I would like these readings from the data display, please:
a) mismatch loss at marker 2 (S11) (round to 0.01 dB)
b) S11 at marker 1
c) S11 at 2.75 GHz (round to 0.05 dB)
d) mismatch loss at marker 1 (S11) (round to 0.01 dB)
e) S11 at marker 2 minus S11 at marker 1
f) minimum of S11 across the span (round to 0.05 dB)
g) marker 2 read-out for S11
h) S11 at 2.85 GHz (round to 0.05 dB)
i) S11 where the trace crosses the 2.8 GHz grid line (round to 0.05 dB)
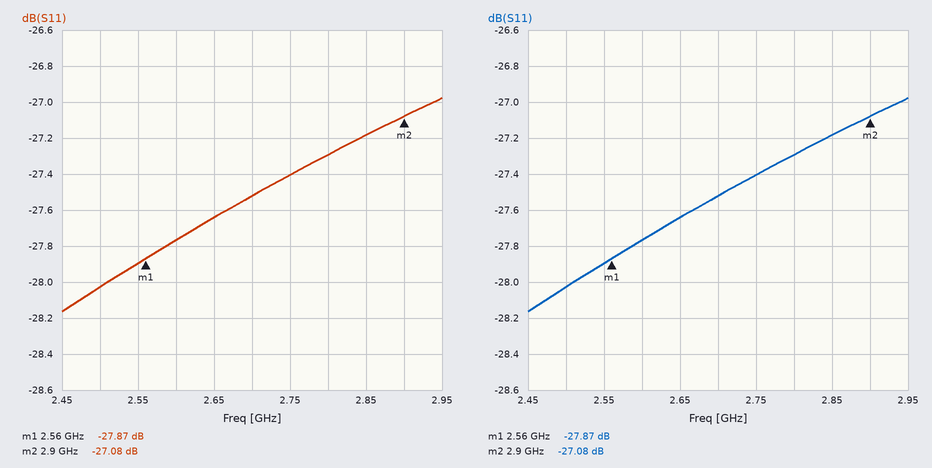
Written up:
0.01 dB
-27.87 dB
-27.40 dB
0.01 dB
0.79 dB
-28.15 dB
-27.08 dB
-27.20 dB
-27.30 dB
